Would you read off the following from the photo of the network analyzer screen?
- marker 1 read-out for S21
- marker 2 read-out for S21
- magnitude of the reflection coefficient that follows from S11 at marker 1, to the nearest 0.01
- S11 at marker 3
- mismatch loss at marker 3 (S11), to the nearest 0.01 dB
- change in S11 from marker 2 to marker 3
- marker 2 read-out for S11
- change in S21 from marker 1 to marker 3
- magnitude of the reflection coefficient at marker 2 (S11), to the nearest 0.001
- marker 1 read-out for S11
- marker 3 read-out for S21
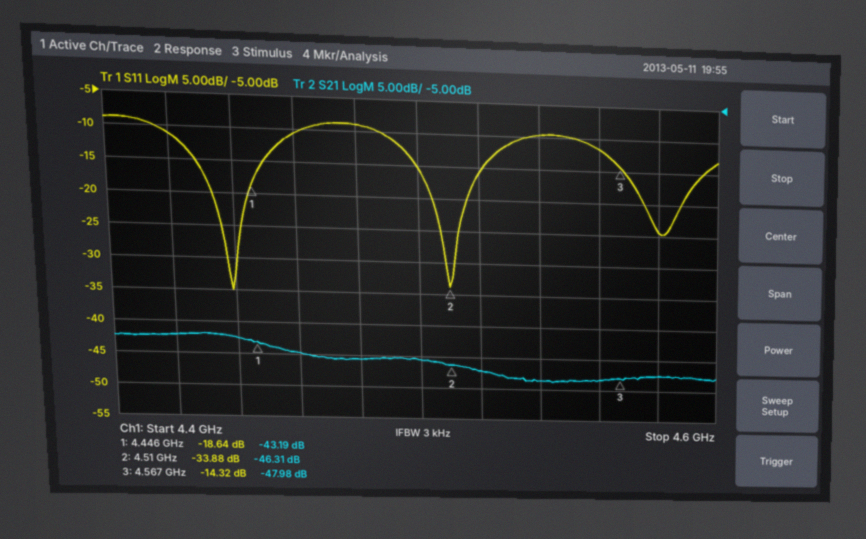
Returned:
-43.19 dB
-46.31 dB
0.12
-14.32 dB
0.16 dB
19.56 dB
-33.88 dB
-4.79 dB
0.020
-18.64 dB
-47.98 dB
